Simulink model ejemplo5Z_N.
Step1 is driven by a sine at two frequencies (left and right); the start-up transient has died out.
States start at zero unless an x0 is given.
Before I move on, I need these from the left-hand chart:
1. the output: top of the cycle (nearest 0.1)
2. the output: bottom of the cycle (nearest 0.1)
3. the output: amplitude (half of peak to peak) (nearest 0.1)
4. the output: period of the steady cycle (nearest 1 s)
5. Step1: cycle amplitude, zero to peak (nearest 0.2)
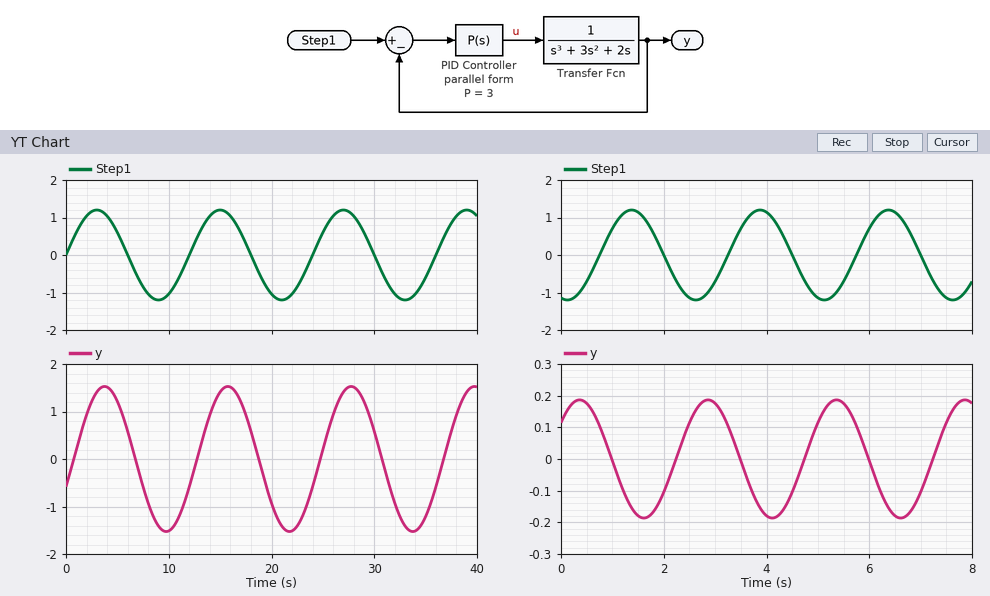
1.5
-1.5
1.5
12 s
1.2
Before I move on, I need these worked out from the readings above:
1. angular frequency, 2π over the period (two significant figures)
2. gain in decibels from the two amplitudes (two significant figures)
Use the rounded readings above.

0.52 rad/s
1.9 dB
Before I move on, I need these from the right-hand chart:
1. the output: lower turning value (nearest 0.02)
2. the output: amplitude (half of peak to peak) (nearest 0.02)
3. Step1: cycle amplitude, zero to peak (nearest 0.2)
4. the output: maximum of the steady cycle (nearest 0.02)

-0.18
0.18
1.2
0.18
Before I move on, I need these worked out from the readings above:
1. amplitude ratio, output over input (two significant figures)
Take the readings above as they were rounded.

0.15
